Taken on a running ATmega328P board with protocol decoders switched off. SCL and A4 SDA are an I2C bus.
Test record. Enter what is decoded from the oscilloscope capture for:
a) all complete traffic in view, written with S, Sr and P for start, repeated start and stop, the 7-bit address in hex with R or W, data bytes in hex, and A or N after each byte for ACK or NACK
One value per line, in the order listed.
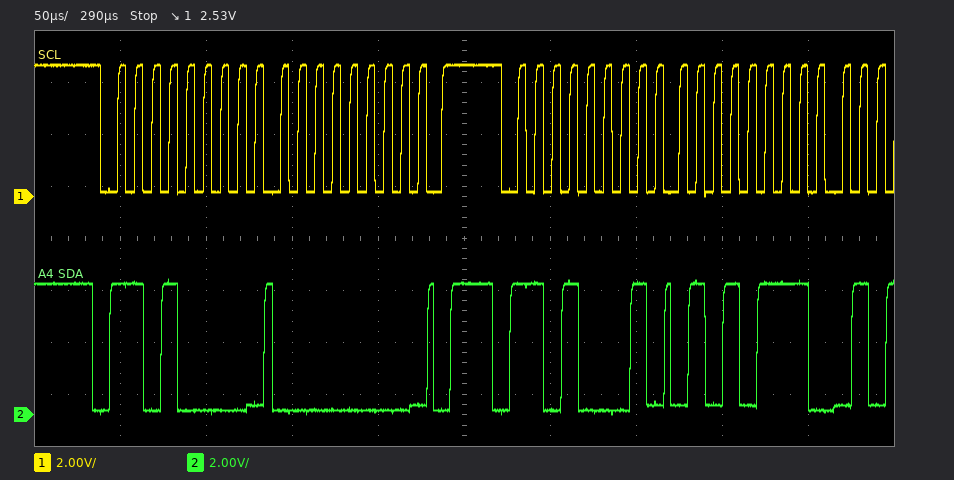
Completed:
S 68W A 00 A P S 68R A 57 A
